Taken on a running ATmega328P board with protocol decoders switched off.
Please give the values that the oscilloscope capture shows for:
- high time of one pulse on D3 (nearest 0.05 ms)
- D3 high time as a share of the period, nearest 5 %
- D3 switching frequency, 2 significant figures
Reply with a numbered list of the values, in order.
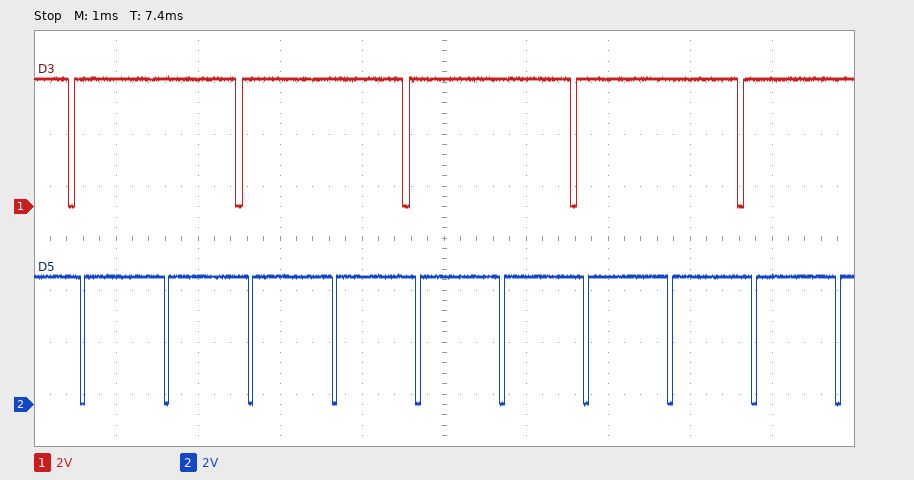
1. 1.95 ms
2. 95 %
3. 490 Hz
